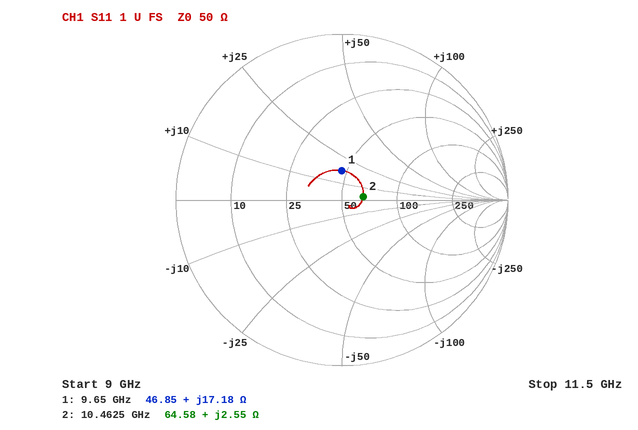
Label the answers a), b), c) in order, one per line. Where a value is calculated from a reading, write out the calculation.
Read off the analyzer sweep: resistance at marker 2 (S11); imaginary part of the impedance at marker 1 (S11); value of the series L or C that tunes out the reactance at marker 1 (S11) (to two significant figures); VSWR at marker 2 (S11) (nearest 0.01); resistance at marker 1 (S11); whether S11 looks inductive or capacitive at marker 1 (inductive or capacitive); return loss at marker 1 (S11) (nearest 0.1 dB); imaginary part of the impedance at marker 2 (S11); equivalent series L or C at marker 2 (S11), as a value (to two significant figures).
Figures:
a) 64.58 Ω
b) +17.18 Ω
c) C = 1/(2π × 9.65 GHz × 17.18 Ω) ≈ 960 fF
d) 1.30
e) 46.85 Ω
f) inductive
g) 15.0 dB
h) +2.55 Ω
i) L = 2.55 Ω/(2π × 10.4625 GHz) ≈ 39 pH
